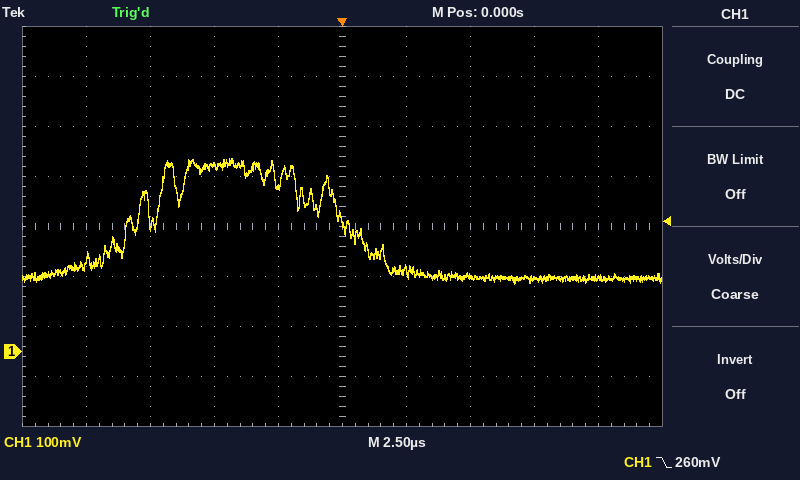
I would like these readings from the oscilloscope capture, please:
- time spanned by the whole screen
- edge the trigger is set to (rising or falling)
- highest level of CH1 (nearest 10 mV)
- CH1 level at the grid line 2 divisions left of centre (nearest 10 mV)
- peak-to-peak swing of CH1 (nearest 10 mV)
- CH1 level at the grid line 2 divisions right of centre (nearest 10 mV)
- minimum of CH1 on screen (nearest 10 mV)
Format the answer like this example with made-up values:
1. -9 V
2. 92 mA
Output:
1. 25 µs
2. falling
3. 390 mV
4. 370 mV
5. 250 mV
6. 150 mV
7. 140 mV
